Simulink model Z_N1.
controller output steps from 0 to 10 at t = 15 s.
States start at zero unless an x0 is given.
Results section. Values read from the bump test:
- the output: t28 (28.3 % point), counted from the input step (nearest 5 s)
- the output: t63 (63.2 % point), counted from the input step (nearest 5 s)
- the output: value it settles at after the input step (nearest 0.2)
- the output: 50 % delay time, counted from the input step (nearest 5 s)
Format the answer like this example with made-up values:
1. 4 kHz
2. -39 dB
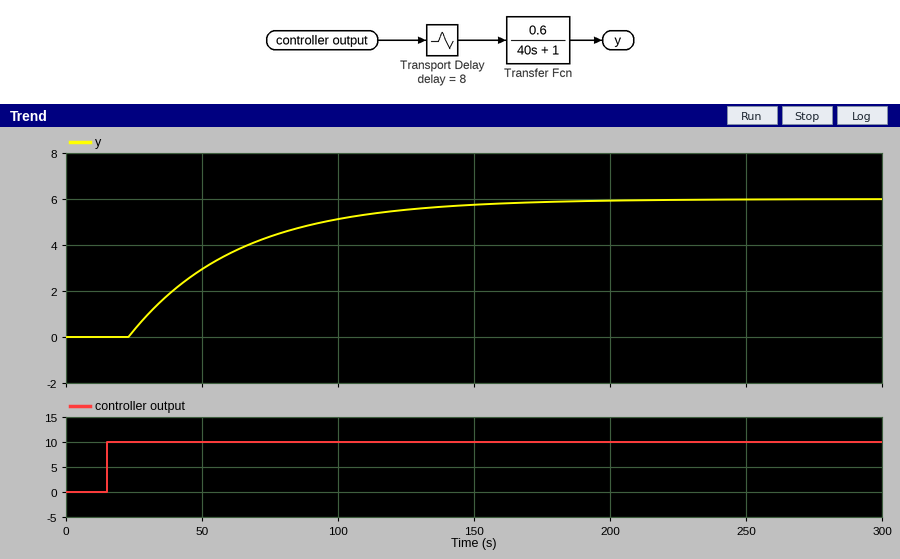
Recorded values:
1. 20 s
2. 50 s
3. 6.0
4. 35 s
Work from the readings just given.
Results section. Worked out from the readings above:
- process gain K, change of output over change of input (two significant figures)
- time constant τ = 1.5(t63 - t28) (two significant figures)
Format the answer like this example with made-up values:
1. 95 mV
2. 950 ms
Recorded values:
1. 0.60
2. 45 s
